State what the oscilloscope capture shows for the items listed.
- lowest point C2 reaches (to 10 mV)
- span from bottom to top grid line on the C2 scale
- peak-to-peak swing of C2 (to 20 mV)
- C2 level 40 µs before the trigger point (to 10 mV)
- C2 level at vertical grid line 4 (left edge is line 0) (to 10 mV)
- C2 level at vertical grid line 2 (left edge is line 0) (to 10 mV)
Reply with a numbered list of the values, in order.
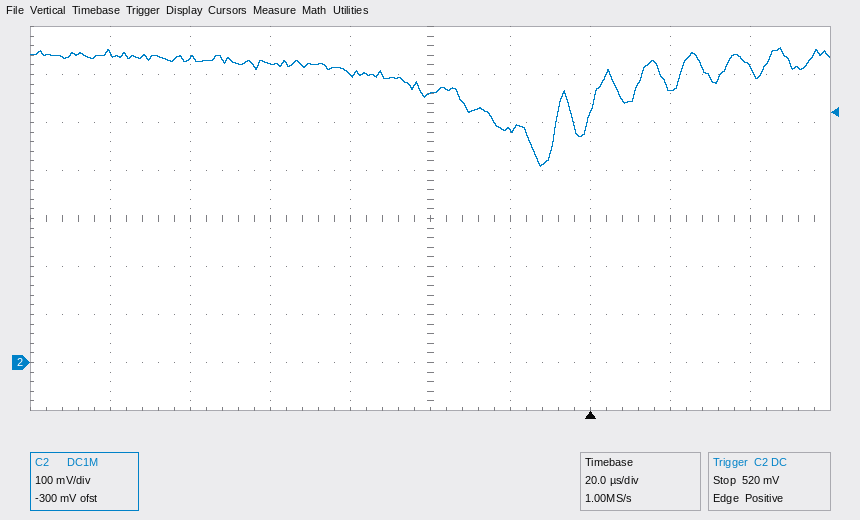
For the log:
1. 410 mV
2. 800 mV
3. 240 mV
4. 560 mV
5. 600 mV
6. 630 mV
